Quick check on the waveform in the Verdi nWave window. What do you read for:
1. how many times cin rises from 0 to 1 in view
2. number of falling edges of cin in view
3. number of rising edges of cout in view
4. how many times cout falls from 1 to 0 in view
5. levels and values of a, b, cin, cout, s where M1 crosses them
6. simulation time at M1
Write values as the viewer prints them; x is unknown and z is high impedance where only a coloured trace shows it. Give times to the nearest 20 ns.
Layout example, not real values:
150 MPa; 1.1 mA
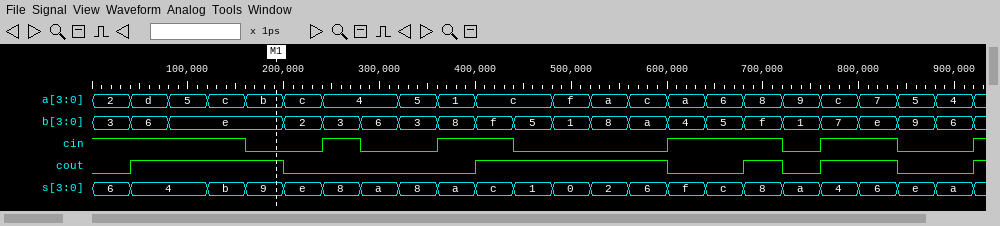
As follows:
5; 5; 5; 4; a=b, b=e, cin=0, cout=1, s=9; 200 ns
